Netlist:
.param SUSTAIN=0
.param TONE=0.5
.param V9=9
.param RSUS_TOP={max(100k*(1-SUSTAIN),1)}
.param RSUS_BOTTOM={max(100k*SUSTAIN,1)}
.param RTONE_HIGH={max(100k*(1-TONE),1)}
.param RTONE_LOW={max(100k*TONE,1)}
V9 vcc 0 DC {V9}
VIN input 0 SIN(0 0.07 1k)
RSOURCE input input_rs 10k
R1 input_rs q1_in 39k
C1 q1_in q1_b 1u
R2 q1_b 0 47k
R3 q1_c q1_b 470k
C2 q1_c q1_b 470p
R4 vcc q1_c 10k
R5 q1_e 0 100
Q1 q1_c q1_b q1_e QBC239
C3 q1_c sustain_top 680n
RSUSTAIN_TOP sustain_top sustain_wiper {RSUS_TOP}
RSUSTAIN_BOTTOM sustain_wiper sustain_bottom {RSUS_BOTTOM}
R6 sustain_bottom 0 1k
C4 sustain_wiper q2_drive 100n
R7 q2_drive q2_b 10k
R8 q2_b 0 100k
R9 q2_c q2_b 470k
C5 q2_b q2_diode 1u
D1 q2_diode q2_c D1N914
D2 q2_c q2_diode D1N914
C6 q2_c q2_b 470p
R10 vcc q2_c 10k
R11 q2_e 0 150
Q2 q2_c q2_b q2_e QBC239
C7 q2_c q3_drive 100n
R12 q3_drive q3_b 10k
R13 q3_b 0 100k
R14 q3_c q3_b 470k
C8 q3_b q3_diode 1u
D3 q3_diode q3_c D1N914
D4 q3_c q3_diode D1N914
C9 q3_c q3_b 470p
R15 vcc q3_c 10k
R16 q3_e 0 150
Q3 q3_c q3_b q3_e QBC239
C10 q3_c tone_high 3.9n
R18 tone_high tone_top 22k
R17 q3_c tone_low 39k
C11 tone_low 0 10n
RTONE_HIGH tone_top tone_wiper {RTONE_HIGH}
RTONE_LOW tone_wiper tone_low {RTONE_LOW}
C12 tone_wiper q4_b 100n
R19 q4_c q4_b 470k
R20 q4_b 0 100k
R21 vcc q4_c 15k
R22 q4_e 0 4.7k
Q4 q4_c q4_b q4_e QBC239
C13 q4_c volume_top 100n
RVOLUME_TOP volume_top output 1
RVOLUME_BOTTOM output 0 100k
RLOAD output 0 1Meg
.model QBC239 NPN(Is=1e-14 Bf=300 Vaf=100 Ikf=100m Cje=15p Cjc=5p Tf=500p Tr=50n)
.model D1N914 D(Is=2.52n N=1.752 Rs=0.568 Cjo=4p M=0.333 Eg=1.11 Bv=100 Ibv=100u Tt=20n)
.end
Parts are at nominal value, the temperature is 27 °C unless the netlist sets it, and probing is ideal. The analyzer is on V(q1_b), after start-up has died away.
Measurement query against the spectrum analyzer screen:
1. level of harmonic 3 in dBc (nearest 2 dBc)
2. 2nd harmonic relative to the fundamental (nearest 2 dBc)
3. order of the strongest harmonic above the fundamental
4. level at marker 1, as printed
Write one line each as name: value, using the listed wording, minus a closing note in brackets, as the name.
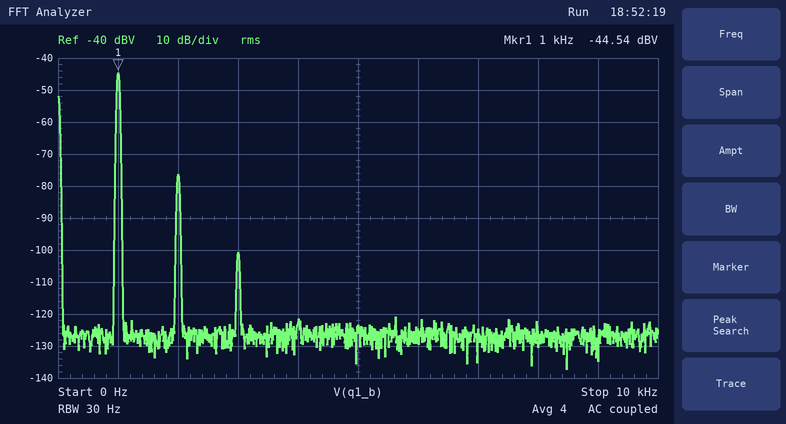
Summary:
level of harmonic 3 in dBc: -56 dBc
2nd harmonic relative to the fundamental: -32 dBc
order of the strongest harmonic above the fundamental: 2
level at marker 1, as printed: -44.54 dBV
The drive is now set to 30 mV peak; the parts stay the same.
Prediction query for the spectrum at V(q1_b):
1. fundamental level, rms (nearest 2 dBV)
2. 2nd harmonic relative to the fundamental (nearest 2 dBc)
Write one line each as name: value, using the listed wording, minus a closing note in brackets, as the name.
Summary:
fundamental level, rms: -52 dBV
2nd harmonic relative to the fundamental: -40 dBc
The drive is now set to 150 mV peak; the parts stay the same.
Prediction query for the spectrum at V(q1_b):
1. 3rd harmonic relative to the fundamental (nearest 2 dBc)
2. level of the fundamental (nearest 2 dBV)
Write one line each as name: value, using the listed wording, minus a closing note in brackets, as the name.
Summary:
3rd harmonic relative to the fundamental: -42 dBc
level of the fundamental: -38 dBV
